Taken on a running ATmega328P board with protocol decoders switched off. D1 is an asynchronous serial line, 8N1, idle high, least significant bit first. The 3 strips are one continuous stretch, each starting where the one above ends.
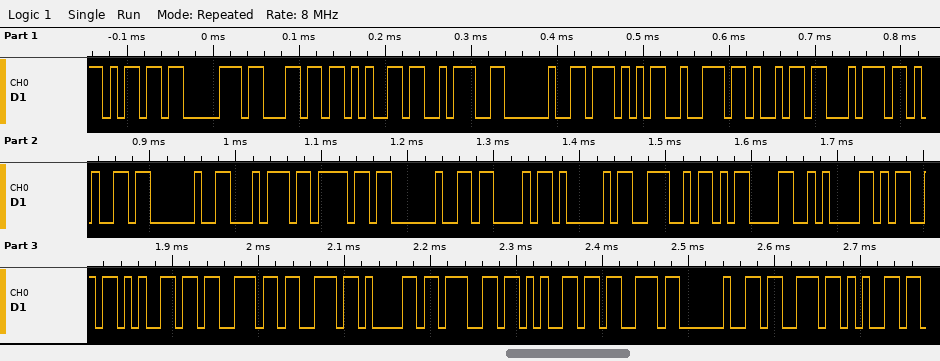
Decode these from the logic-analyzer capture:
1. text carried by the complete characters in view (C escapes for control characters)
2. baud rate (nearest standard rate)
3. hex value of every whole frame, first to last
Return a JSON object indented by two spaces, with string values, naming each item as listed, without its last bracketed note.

{
  "text carried by the complete characters in view": "\"mple: Write to CAN\\r\\nMessages se\"",
  "baud rate": "115200 baud",
  "hex value of every whole frame, first to last": "6D 70 6C 65 3A 20 57 72 69 74 65 20 74 6F 20 43 41 4E 0D 0A 4D 65 73 73 61 67 65 73 20 73 65"
}
